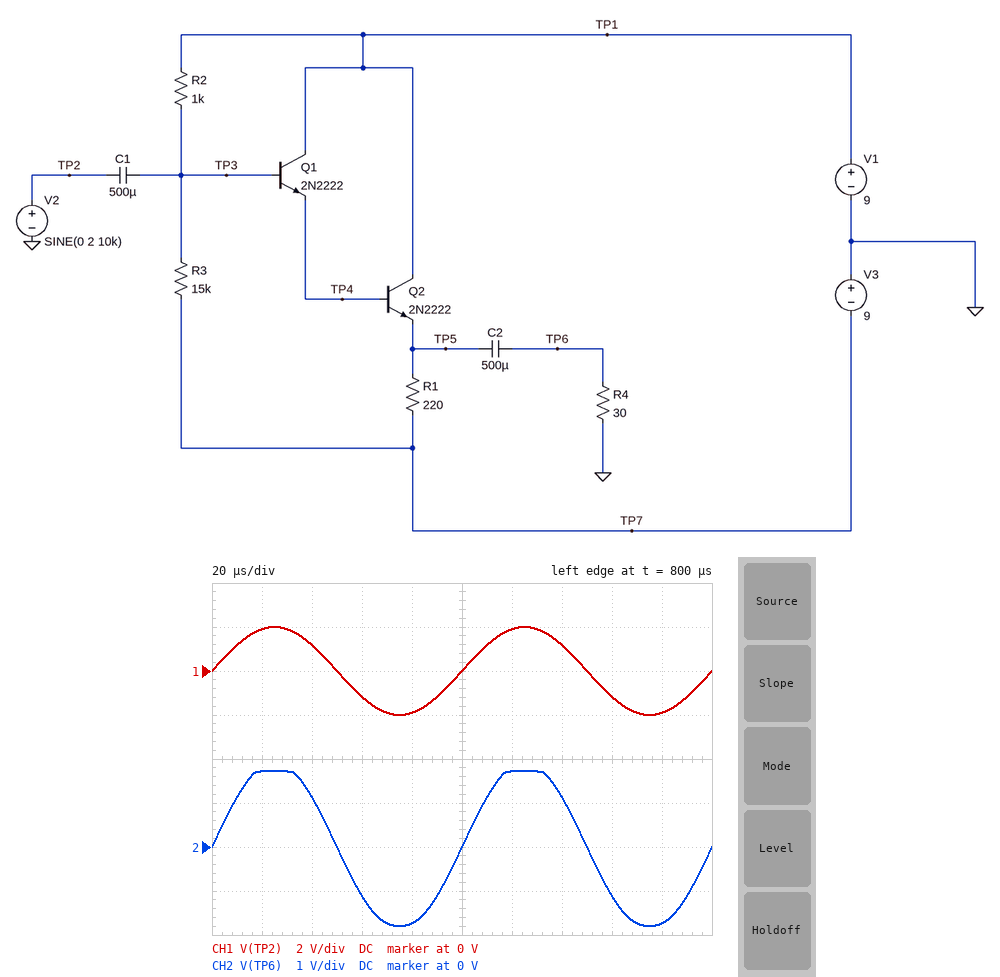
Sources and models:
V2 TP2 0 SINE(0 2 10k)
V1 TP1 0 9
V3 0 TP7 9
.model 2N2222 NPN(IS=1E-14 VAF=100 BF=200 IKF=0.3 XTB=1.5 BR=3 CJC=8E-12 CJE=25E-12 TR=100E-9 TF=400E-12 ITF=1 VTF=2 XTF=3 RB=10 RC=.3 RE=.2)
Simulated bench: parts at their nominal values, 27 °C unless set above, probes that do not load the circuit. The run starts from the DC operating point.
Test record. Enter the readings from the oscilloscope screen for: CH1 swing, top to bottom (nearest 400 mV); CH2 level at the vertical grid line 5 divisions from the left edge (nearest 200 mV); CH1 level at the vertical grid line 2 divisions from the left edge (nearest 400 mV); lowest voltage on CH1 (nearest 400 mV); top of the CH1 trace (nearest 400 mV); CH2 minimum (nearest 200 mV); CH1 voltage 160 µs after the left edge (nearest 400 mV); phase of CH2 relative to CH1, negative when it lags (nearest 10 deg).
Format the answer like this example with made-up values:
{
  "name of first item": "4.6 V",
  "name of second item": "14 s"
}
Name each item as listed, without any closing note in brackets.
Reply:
{
  "CH1 swing, top to bottom": "4.0 V",
  "CH2 level at the vertical grid line 5 divisions from the left edge": "0 V",
  "CH1 level at the vertical grid line 2 divisions from the left edge": "1.2 V",
  "lowest voltage on CH1": "-2.0 V",
  "top of the CH1 trace": "2.0 V",
  "CH2 minimum": "-1.8 V",
  "CH1 voltage 160 µs after the left edge": "-1.2 V",
  "phase of CH2 relative to CH1, negative when it lags": "0 deg"
}
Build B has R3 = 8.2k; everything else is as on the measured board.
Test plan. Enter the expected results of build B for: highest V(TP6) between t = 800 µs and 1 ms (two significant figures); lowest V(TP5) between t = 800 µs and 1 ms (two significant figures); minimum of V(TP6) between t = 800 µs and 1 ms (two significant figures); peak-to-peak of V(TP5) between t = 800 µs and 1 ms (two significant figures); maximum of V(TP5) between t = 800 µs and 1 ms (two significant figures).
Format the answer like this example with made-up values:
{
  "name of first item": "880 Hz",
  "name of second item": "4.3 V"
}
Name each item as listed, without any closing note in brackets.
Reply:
{
  "highest V(TP6) between t = 800 µs and 1 ms": "1.9 V",
  "lowest V(TP5) between t = 800 µs and 1 ms": "3.9 V",
  "minimum of V(TP6) between t = 800 µs and 1 ms": "-1.7 V",
  "peak-to-peak of V(TP5) between t = 800 µs and 1 ms": "3.7 V",
  "maximum of V(TP5) between t = 800 µs and 1 ms": "7.6 V"
}
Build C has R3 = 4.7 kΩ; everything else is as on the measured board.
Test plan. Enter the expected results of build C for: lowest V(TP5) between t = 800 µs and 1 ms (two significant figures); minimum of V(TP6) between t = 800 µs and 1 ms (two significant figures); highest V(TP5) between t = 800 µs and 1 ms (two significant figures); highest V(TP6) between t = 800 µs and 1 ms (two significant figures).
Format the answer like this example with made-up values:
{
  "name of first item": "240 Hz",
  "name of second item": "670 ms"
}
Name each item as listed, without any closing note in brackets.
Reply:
{
  "lowest V(TP5) between t = 800 µs and 1 ms": "2.8 V",
  "minimum of V(TP6) between t = 800 µs and 1 ms": "-1.6 V",
  "highest V(TP5) between t = 800 µs and 1 ms": "6.4 V",
  "highest V(TP6) between t = 800 µs and 1 ms": "1.9 V"
}
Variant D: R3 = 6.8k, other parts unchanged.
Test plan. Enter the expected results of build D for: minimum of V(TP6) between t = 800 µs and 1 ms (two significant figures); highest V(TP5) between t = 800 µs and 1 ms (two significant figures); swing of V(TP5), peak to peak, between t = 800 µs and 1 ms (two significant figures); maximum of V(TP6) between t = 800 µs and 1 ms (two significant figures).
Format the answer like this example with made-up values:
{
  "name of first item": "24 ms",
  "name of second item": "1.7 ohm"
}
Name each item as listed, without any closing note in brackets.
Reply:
{
  "minimum of V(TP6) between t = 800 µs and 1 ms": "-1.7 V",
  "highest V(TP5) between t = 800 µs and 1 ms": "7.2 V",
  "swing of V(TP5), peak to peak, between t = 800 µs and 1 ms": "3.6 V",
  "maximum of V(TP6) between t = 800 µs and 1 ms": "1.9 V"
}
